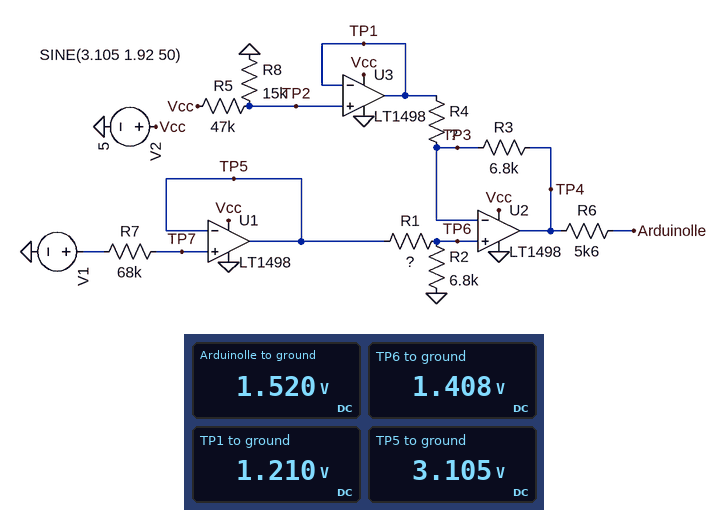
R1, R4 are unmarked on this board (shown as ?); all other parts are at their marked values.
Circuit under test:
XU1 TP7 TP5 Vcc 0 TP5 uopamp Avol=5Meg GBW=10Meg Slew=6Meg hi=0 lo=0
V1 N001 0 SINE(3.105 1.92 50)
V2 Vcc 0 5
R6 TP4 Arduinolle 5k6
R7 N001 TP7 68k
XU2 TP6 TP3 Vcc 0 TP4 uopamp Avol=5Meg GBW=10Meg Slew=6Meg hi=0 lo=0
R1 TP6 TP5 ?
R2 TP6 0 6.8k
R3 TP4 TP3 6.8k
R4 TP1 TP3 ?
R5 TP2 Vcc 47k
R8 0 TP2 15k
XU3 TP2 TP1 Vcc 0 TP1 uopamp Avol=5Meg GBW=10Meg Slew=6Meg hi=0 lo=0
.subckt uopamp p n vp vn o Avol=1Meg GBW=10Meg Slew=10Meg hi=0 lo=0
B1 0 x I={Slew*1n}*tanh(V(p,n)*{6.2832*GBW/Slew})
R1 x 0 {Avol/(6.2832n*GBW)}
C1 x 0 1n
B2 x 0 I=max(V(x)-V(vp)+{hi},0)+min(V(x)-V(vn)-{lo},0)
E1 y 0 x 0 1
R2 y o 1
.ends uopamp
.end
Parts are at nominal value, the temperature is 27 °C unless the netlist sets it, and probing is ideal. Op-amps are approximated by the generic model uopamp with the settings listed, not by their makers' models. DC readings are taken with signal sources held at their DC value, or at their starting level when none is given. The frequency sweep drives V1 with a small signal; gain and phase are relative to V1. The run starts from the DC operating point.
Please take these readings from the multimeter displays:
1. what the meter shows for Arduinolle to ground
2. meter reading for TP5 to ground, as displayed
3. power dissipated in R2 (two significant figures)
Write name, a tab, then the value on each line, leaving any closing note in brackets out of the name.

what the meter shows for Arduinolle to ground	1.520 V
meter reading for TP5 to ground, as displayed	3.105 V
power dissipated in R2	290 µW
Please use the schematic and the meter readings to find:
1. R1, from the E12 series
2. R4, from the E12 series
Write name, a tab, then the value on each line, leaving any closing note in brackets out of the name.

R1, from the E12 series	8.2 kΩ
R4, from the E12 series	12 kΩ
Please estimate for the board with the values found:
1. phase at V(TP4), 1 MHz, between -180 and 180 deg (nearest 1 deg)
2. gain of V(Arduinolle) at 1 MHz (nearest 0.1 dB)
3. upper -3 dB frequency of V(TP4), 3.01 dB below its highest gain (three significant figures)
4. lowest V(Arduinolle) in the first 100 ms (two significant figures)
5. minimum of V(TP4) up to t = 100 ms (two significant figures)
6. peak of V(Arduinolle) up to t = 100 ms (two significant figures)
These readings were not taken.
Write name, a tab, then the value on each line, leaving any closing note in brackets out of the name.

phase at V(TP4), 1 MHz, between -180 and 180 deg	-15 deg
gain of V(Arduinolle) at 1 MHz	-3.1 dB
upper -3 dB frequency of V(TP4), 3.01 dB below its highest gain	4.96 MHz
lowest V(Arduinolle) in the first 100 ms	160 mV
minimum of V(TP4) up to t = 100 ms	160 mV
peak of V(Arduinolle) up to t = 100 ms	2.9 V
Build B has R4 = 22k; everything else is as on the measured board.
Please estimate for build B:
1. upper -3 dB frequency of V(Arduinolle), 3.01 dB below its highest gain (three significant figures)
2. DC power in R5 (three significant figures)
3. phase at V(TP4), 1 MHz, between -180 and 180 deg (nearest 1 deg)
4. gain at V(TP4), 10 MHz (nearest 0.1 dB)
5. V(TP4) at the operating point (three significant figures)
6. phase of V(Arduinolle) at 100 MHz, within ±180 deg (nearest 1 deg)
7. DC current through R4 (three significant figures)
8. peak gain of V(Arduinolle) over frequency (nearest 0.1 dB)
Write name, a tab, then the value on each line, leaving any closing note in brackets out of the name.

upper -3 dB frequency of V(Arduinolle), 3.01 dB below its highest gain	5.55 MHz
DC power in R5	306 µW
phase at V(TP4), 1 MHz, between -180 and 180 deg	-13 deg
gain at V(TP4), 10 MHz	-11.9 dB
V(TP4) at the operating point	1.47 V
phase of V(Arduinolle) at 100 MHz, within ±180 deg	-170 deg
DC current through R4	9.00 µA
peak gain of V(Arduinolle) over frequency	-4.5 dB
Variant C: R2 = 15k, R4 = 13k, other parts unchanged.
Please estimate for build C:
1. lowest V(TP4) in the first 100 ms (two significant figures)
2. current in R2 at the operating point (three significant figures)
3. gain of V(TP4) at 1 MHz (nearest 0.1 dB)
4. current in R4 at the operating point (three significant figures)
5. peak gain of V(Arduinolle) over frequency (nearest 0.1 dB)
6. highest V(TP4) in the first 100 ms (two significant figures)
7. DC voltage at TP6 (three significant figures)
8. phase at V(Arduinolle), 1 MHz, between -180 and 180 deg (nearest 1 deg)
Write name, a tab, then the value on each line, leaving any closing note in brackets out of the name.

lowest V(TP4) in the first 100 ms	530 mV
current in R2 at the operating point	134 µA
gain of V(TP4) at 1 MHz	-0.3 dB
current in R4 at the operating point	61.4 µA
peak gain of V(Arduinolle) over frequency	-0.1 dB
highest V(TP4) in the first 100 ms	4.3 V
DC voltage at TP6	2.01 V
phase at V(Arduinolle), 1 MHz, between -180 and 180 deg	-14 deg
